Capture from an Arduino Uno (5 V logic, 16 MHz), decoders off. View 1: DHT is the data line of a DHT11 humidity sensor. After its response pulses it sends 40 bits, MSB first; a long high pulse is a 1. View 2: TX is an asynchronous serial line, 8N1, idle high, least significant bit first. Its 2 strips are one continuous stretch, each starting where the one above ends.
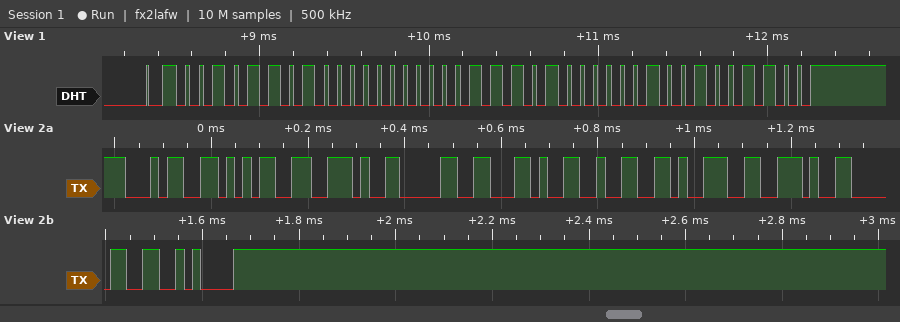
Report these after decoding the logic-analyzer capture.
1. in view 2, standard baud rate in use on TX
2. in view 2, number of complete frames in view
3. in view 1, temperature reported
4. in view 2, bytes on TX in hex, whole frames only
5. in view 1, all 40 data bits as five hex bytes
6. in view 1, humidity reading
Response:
57600 baud
10
29.2 °C
34 35 2E 30 2C 32 39 2E 30 0A
2D 00 1D 02 4C
45 %
